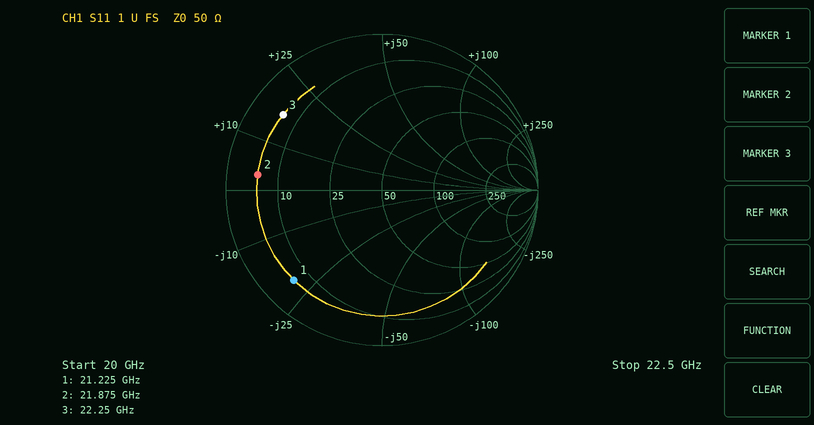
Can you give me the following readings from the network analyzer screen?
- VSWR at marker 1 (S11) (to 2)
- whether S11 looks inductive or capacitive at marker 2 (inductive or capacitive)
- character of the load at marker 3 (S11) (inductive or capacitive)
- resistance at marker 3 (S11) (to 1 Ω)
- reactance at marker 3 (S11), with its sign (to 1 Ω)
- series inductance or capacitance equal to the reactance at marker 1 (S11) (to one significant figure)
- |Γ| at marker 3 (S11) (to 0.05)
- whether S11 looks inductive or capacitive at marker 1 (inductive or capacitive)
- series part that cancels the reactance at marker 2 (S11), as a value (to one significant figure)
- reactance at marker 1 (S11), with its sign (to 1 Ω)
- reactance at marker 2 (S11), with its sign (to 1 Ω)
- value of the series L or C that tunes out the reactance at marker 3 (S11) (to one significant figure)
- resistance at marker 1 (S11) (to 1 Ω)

10
inductive
inductive
6 Ω
+17 Ω
400 fF
0.80
capacitive
2 pF
-21 Ω
+3 Ω
400 fF
6 Ω
